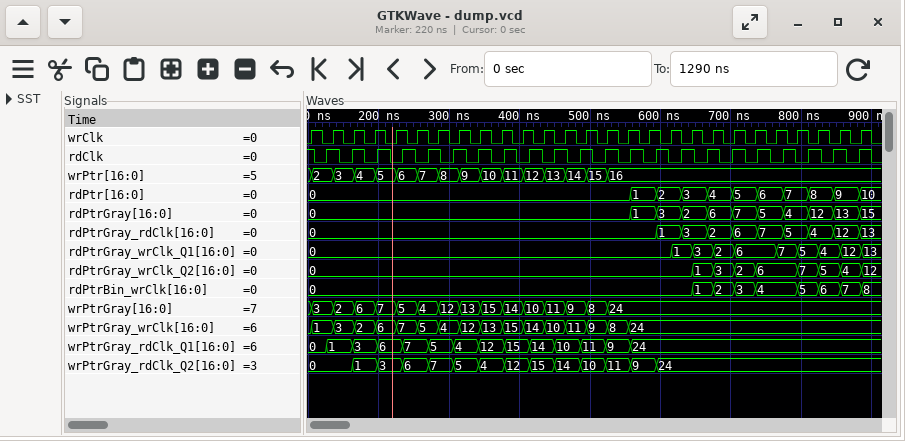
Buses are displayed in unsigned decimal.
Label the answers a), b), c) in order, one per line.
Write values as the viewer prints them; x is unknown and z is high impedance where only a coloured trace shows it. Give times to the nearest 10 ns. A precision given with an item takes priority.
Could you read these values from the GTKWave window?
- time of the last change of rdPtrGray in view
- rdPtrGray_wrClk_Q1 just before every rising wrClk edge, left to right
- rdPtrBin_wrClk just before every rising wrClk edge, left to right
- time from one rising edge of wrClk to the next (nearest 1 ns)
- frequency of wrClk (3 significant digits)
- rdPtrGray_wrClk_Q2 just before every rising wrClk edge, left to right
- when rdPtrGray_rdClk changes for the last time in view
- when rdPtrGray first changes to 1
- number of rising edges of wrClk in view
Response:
a) 880 ns
b) 0, 0, 0, 0, 0, 0, 0, 0, 0, 0, 0, 0, 0, 0, 0, 0, 0, 0, 1, 3, 2, 6, 6, 7, 5, 4, 12
c) 0, 0, 0, 0, 0, 0, 0, 0, 0, 0, 0, 0, 0, 0, 0, 0, 0, 0, 0, 1, 2, 3, 4, 4, 5, 6, 7
d) 30 ns
e) 33.3 MHz
f) 0, 0, 0, 0, 0, 0, 0, 0, 0, 0, 0, 0, 0, 0, 0, 0, 0, 0, 0, 1, 3, 2, 6, 6, 7, 5, 4
g) 880 ns
h) 560 ns
i) 27
